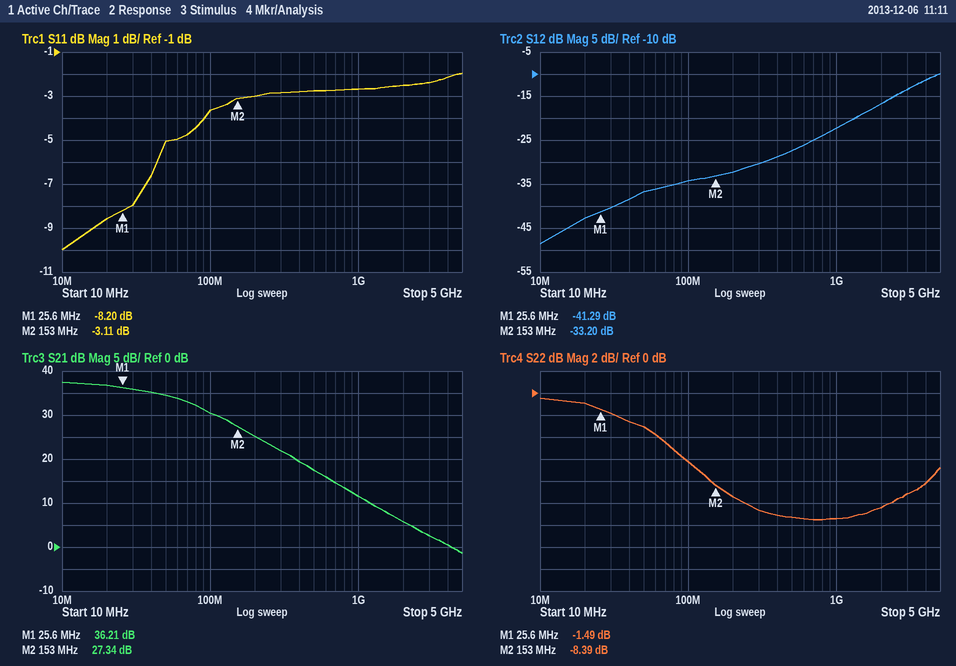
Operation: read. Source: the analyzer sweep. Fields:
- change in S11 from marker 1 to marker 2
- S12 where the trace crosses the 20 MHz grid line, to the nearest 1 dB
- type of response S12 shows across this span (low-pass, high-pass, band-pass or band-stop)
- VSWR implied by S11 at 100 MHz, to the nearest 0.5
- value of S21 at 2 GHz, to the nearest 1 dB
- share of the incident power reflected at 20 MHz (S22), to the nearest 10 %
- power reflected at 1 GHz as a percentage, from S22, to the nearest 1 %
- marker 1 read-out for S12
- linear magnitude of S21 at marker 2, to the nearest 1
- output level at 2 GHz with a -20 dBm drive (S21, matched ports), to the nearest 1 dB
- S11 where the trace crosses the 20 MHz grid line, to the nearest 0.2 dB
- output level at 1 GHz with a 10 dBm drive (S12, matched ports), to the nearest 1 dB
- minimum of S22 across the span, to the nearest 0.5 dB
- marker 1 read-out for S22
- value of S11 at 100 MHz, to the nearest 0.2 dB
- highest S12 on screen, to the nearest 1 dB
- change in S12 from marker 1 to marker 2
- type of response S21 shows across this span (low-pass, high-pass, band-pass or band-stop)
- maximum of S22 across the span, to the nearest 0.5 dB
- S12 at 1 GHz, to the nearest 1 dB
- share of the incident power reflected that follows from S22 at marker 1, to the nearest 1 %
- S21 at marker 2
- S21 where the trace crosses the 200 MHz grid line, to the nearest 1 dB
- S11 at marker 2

5.09 dB
-43 dB
high-pass
5.0
6 dB
80 %
7 %
-41.29 dB
23
-14 dBm
-8.6 dB
-12 dBm
-11.5 dB
-1.49 dB
-3.6 dB
-10 dB
8.09 dB
low-pass
-0.5 dB
-22 dB
71 %
27.34 dB
25 dB
-3.11 dB
